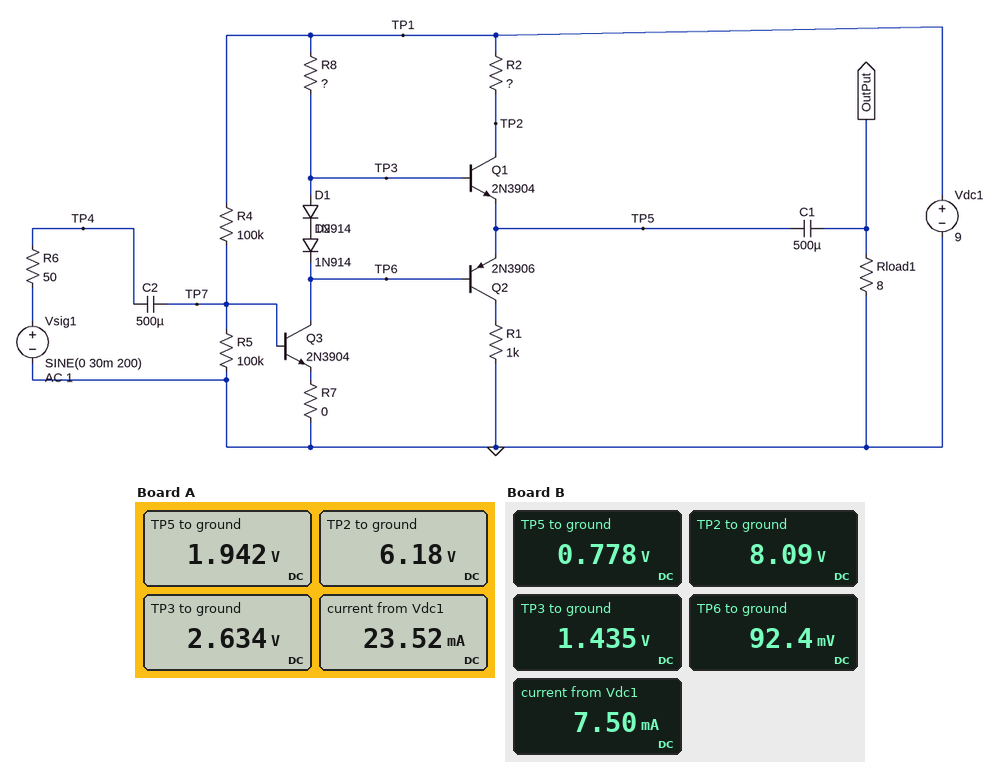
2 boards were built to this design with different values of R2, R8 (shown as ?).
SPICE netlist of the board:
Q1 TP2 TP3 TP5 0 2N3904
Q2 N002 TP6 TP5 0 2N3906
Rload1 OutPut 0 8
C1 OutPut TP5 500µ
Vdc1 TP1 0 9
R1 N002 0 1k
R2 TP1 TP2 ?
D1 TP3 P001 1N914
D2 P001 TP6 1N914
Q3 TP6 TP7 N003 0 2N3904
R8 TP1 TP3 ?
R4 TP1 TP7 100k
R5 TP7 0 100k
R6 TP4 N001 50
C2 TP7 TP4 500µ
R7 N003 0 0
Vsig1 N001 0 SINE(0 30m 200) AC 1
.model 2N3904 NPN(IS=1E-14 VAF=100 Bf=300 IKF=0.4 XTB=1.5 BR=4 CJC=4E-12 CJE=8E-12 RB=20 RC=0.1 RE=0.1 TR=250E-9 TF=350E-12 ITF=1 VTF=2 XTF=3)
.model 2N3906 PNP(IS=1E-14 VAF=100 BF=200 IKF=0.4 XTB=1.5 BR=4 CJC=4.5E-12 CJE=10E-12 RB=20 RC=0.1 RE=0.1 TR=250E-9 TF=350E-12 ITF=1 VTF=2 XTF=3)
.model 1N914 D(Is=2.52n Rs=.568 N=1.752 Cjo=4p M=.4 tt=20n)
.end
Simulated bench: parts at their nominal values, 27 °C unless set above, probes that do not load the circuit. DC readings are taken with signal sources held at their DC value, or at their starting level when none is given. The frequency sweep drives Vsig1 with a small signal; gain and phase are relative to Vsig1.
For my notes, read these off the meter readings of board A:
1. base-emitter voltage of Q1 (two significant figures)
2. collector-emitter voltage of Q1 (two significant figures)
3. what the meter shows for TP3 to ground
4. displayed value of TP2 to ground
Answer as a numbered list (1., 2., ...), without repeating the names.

1. 690 mV
2. 4.2 V
3. 2.634 V
4. 6.18 V
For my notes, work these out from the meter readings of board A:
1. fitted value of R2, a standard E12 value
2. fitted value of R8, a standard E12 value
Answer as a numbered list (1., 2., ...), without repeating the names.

1. 680 Ω
2. 330 Ω
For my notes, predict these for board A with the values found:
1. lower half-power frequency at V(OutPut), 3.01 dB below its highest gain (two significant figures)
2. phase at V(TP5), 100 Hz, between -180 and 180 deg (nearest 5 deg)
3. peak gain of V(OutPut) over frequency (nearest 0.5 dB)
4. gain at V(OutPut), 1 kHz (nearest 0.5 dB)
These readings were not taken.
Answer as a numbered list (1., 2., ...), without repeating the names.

1. 5.5 Hz
2. 160 deg
3. 26.5 dB
4. 26.5 dB
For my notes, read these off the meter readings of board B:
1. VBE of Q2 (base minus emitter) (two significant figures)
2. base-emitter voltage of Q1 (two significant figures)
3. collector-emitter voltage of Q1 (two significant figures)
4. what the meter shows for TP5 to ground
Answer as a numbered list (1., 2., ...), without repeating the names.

1. -690 mV
2. 660 mV
3. 7.3 V
4. 0.778 V
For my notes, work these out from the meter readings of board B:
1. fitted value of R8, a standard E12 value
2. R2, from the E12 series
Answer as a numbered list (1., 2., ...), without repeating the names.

1. 1.2 kΩ
2. 820 Ω
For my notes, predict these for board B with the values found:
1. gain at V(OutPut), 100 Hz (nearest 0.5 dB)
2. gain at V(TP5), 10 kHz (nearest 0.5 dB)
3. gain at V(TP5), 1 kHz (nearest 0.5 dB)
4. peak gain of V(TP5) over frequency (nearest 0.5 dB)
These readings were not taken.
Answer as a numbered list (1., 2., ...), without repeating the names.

1. 2.0 dB
2. 2.0 dB
3. 2.0 dB
4. 12.0 dB
